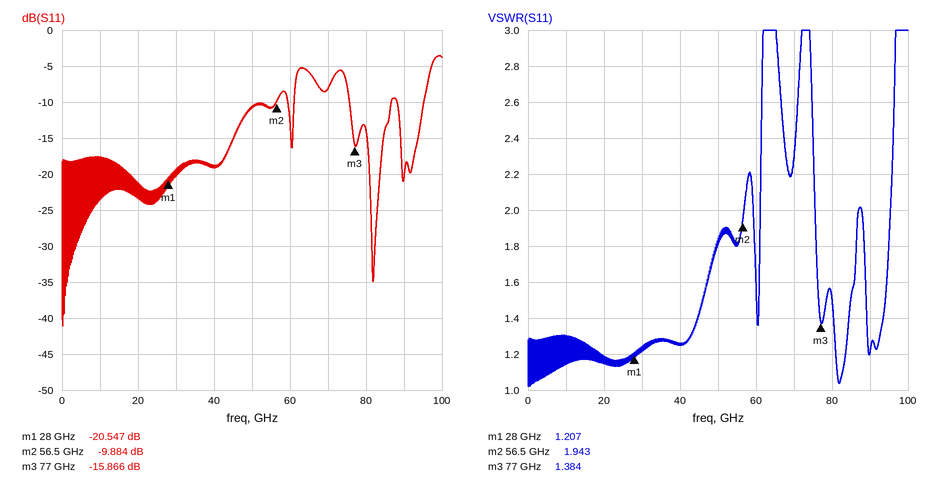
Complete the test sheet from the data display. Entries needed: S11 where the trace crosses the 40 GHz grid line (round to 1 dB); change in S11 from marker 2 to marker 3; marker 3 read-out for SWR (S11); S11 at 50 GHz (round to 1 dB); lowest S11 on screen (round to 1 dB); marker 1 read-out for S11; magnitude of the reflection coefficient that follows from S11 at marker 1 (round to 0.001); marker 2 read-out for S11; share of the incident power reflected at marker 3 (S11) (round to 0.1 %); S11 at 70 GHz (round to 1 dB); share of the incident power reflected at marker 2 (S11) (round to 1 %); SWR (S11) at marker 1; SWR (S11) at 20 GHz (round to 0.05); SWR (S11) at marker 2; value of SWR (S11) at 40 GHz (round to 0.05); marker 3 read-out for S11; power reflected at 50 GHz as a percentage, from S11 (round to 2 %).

-19 dB
-5.982 dB
1.384
-11 dB
-41 dB
-20.547 dB
0.094
-9.884 dB
2.6 %
-8 dB
10 %
1.207
1.15
1.943
1.25
-15.866 dB
8 %
